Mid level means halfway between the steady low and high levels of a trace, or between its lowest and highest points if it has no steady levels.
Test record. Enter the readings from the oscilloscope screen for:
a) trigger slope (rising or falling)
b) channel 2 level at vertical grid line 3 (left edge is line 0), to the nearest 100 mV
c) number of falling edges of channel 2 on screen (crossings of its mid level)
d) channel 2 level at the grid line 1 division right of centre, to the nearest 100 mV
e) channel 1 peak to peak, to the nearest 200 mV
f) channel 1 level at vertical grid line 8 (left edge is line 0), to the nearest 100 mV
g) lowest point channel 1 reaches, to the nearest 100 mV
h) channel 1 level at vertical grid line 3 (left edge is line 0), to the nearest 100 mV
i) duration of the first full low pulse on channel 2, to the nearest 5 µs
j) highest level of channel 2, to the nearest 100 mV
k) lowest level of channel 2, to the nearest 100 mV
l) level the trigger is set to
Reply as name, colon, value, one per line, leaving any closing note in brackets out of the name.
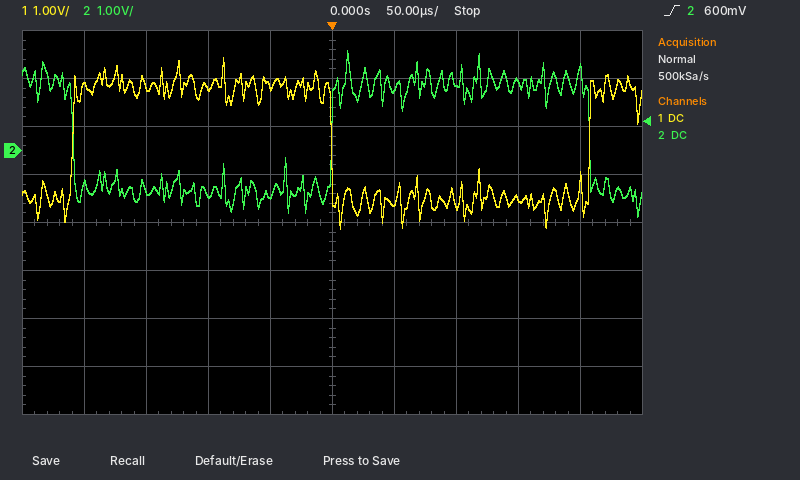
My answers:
trigger slope: rising
channel 2 level at vertical grid line 3 (left edge is line 0), to the nearest 100 mV: -900 mV
number of falling edges of channel 2 on screen: 2
channel 2 level at the grid line 1 division right of centre, to the nearest 100 mV: 1.3 V
channel 1 peak to peak, to the nearest 200 mV: 3.6 V
channel 1 level at vertical grid line 8 (left edge is line 0), to the nearest 100 mV: -1.0 V
lowest point channel 1 reaches, to the nearest 100 mV: -1.6 V
channel 1 level at vertical grid line 3 (left edge is line 0), to the nearest 100 mV: 1.3 V
duration of the first full low pulse on channel 2, to the nearest 5 µs: 210 µs
highest level of channel 2, to the nearest 100 mV: 2.1 V
lowest level of channel 2, to the nearest 100 mV: -1.4 V
level the trigger is set to: 600 mV
